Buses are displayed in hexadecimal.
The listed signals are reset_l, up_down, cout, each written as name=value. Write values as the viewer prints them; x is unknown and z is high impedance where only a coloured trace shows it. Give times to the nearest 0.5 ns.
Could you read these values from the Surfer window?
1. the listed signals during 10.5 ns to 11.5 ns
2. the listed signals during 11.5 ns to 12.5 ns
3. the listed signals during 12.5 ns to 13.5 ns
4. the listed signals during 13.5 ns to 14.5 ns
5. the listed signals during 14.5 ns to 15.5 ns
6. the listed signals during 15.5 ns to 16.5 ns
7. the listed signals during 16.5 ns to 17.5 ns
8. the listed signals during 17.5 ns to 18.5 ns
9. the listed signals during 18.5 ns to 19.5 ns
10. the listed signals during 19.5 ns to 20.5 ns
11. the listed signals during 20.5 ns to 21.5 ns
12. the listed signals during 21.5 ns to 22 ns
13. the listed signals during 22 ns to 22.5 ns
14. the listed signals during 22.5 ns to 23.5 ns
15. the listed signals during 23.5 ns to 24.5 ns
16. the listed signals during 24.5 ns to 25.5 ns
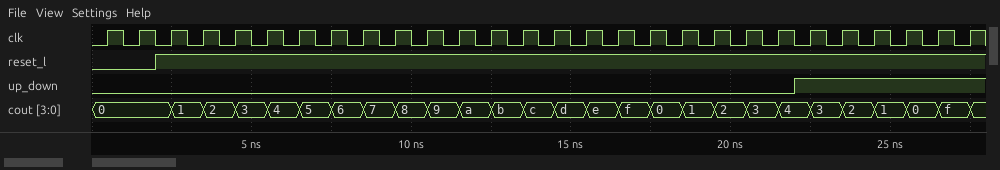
reset_l=1, up_down=0, cout=9
reset_l=1, up_down=0, cout=a
reset_l=1, up_down=0, cout=b
reset_l=1, up_down=0, cout=c
reset_l=1, up_down=0, cout=d
reset_l=1, up_down=0, cout=e
reset_l=1, up_down=0, cout=f
reset_l=1, up_down=0, cout=0
reset_l=1, up_down=0, cout=1
reset_l=1, up_down=0, cout=2
reset_l=1, up_down=0, cout=3
reset_l=1, up_down=0, cout=4
reset_l=1, up_down=1, cout=4
reset_l=1, up_down=1, cout=3
reset_l=1, up_down=1, cout=2
reset_l=1, up_down=1, cout=1
